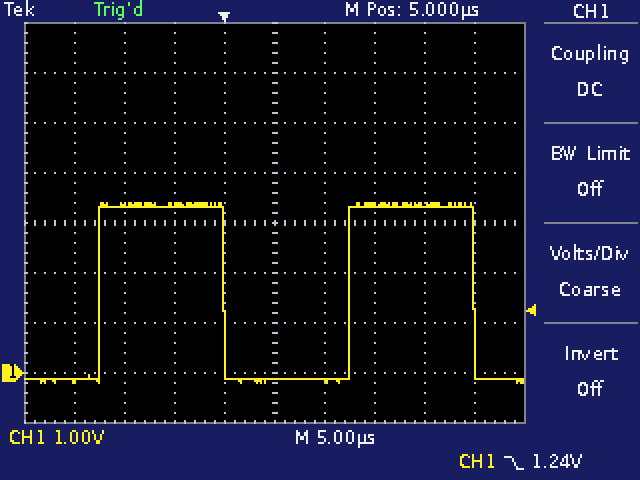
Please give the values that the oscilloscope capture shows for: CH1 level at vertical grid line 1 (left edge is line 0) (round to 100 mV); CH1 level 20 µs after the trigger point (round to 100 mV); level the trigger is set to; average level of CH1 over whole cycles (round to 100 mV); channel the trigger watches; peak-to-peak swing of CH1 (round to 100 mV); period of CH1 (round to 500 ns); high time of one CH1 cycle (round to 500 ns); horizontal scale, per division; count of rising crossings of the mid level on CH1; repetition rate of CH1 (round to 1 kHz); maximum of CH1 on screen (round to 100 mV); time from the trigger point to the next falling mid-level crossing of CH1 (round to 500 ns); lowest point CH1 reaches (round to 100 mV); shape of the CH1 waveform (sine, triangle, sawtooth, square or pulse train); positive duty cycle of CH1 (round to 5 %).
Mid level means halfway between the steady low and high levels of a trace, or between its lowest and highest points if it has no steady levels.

-200 mV
3.4 V
1.24 V
1.6 V
CH1
3.6 V
25.0 µs
12.5 µs
5 µs
2
40 kHz
3.4 V
25.0 µs
-200 mV
square
50 %
